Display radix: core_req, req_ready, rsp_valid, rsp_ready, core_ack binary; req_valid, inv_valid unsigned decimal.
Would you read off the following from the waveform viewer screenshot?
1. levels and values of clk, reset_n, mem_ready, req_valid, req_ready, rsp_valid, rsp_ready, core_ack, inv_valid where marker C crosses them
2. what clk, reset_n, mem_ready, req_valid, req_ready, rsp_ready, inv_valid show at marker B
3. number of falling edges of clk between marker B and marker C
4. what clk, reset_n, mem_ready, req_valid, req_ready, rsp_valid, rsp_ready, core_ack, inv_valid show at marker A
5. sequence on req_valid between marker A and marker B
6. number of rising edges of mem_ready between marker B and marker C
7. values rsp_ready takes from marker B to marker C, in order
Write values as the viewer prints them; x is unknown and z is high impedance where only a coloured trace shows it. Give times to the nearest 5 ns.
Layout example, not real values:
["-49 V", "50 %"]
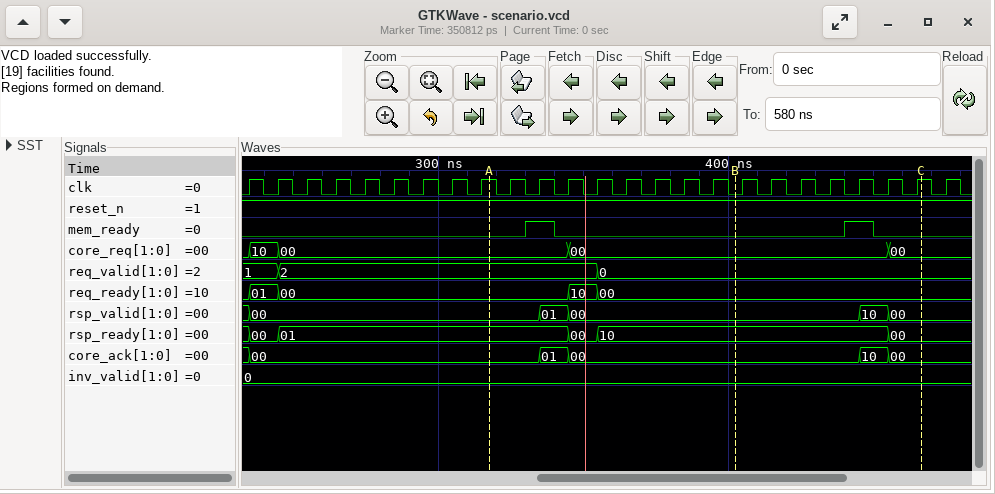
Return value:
["clk=1, reset_n=1, mem_ready=0, req_valid=0, req_ready=00, rsp_valid=00, rsp_ready=00, core_ack=00, inv_valid=0", "clk=0, reset_n=1, mem_ready=0, req_valid=0, req_ready=00, rsp_ready=10, inv_valid=0", "6", "clk=1, reset_n=1, mem_ready=0, req_valid=2, req_ready=00, rsp_valid=00, rsp_ready=01, core_ack=00, inv_valid=0", "2, 0", "1", "10, 00"]
